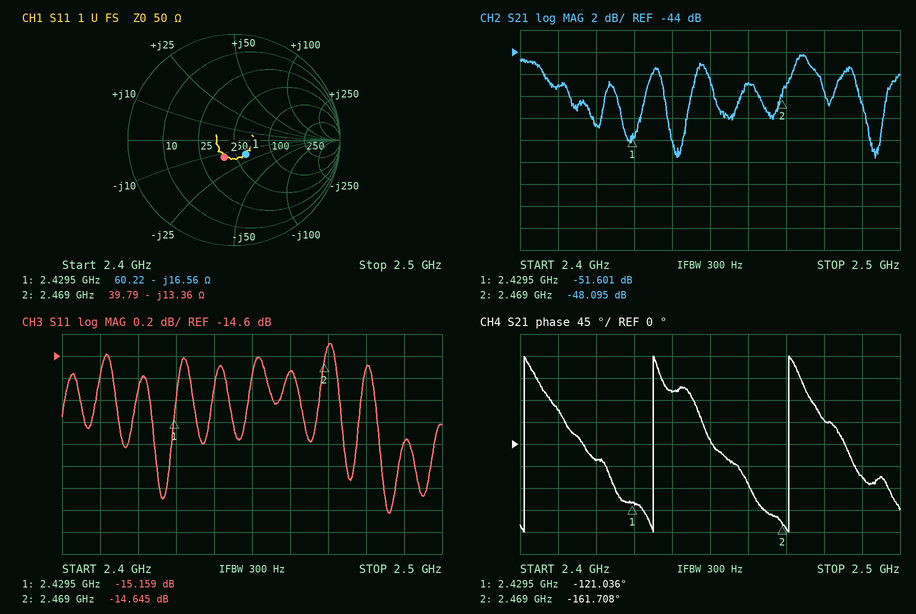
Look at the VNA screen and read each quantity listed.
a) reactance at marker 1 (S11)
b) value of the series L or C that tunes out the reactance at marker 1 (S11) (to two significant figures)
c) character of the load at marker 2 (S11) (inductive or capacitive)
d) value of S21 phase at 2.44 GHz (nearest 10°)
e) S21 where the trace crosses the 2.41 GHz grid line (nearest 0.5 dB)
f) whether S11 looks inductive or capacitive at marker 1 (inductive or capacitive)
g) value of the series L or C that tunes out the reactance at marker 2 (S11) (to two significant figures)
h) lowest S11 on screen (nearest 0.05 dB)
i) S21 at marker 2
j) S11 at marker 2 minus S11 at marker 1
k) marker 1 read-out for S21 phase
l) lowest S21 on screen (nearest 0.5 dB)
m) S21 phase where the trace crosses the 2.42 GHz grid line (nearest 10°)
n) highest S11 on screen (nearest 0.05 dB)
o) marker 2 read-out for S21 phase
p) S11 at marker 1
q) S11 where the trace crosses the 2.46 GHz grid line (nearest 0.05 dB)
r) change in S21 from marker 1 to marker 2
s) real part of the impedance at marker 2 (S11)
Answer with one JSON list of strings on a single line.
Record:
["-16.56 Ω", "1.1 nH", "capacitive", "110°", "-47.0 dB", "capacitive", "860 pH", "-16.05 dB", "-48.095 dB", "0.514 dB", "-121.036°", "-53.5 dB", "-30°", "-14.50 dB", "-161.708°", "-15.159 dB", "-14.75 dB", "3.506 dB", "39.79 Ω"]
